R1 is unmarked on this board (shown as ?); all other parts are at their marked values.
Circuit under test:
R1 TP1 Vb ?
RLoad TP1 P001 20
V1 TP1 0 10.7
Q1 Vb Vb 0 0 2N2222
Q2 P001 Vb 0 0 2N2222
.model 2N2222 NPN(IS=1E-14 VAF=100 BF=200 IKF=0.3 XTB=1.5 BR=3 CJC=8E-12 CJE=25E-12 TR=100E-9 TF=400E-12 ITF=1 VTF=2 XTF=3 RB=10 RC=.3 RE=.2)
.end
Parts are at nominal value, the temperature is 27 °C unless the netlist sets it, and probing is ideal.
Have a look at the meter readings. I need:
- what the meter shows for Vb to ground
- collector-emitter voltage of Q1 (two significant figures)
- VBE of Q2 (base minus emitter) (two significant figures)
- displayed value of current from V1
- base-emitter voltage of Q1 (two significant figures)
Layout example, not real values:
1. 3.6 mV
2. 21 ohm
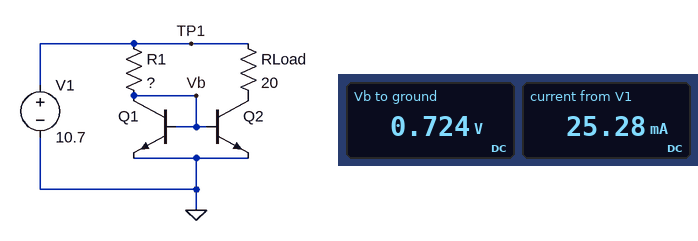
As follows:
1. 0.724 V
2. 720 mV
3. 720 mV
4. 25.28 mA
5. 720 mV
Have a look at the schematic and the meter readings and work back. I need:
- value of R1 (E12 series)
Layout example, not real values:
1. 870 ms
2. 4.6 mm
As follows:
1. 820 Ω
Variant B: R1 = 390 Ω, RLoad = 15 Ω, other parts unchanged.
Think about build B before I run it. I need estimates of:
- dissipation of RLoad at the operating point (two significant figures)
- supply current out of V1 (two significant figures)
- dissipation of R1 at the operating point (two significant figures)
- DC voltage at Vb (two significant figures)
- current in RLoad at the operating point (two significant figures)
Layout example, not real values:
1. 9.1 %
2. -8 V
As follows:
1. 11 mW
2. 53 mA
3. 250 mW
4. 750 mV
5. 27 mA
